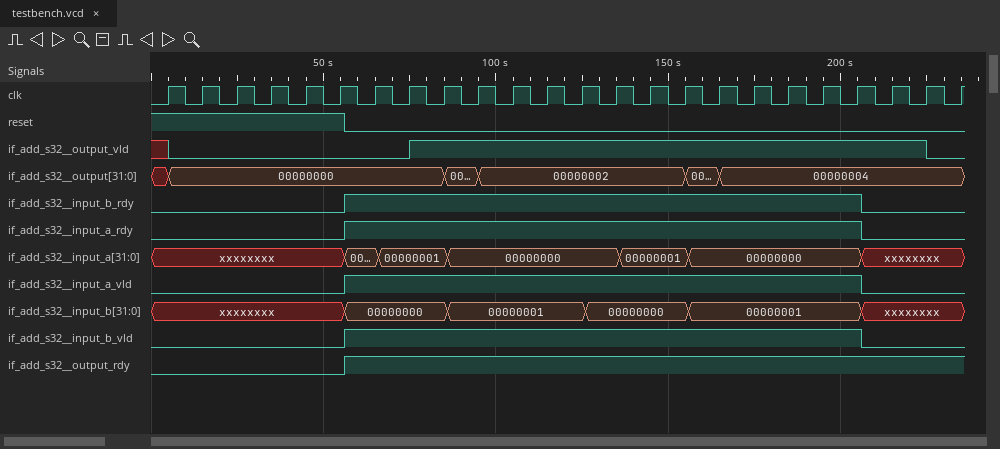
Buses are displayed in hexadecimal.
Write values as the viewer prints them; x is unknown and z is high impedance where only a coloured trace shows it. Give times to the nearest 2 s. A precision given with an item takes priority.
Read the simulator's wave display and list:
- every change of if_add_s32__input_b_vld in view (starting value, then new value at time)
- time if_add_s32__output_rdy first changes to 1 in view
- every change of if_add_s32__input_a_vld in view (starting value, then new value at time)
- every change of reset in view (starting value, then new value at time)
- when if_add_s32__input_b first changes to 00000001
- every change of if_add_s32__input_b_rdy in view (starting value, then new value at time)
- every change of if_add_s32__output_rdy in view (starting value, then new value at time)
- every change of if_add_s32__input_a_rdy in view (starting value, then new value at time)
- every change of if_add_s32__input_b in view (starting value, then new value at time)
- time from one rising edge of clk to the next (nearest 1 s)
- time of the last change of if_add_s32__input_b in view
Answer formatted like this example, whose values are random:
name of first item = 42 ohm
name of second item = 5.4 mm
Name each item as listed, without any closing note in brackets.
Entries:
every change of if_add_s32__input_b_vld in view = 0, 1 at 56 s, 0 at 206 s
time if_add_s32__output_rdy first changes to 1 in view = 56 s
every change of if_add_s32__input_a_vld in view = 0, 1 at 56 s, 0 at 206 s
every change of reset in view = 1, 0 at 56 s
when if_add_s32__input_b first changes to 00000001 = 86 s
every change of if_add_s32__input_b_rdy in view = 0, 1 at 56 s, 0 at 206 s
every change of if_add_s32__output_rdy in view = 0, 1 at 56 s
every change of if_add_s32__input_a_rdy in view = 0, 1 at 56 s, 0 at 206 s
every change of if_add_s32__input_b in view = xxxxxxxx, 00000000 at 56 s, 00000001 at 86 s, 00000000 at 126 s, 00000001 at 156 s, xxxxxxxx at 206 s
time from one rising edge of clk to the next = 10 s
time of the last change of if_add_s32__input_b in view = 206 s
